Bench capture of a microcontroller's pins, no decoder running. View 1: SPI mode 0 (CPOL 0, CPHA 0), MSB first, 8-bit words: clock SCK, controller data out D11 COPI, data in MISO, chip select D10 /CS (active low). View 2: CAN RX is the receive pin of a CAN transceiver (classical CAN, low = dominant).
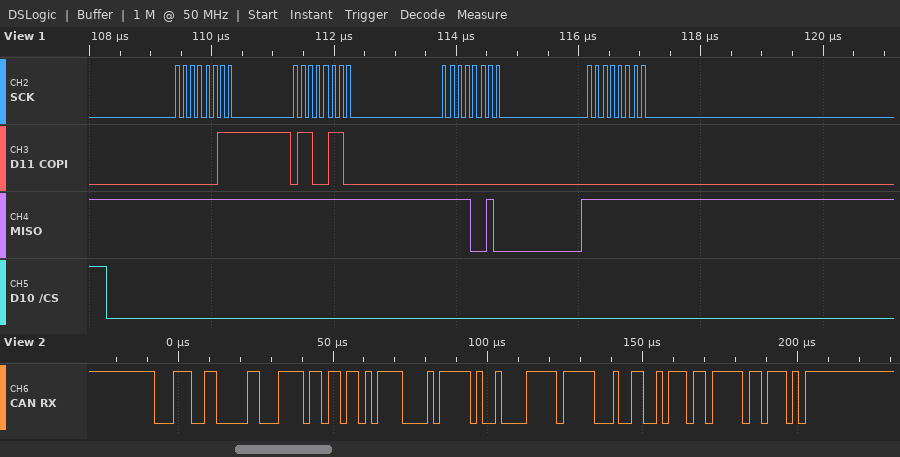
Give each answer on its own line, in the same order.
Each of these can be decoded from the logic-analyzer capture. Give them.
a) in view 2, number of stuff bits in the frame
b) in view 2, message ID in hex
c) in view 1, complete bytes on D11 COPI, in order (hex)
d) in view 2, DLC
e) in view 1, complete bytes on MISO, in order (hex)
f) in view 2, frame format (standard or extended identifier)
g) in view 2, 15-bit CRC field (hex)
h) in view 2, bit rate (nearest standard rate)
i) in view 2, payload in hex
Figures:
5
0x1CC
03 66 00 00
8
FF FF F2 FF
standard
0x6FEE
500 kbit/s
F6 DA F0 BF 21 FF 93 2E
